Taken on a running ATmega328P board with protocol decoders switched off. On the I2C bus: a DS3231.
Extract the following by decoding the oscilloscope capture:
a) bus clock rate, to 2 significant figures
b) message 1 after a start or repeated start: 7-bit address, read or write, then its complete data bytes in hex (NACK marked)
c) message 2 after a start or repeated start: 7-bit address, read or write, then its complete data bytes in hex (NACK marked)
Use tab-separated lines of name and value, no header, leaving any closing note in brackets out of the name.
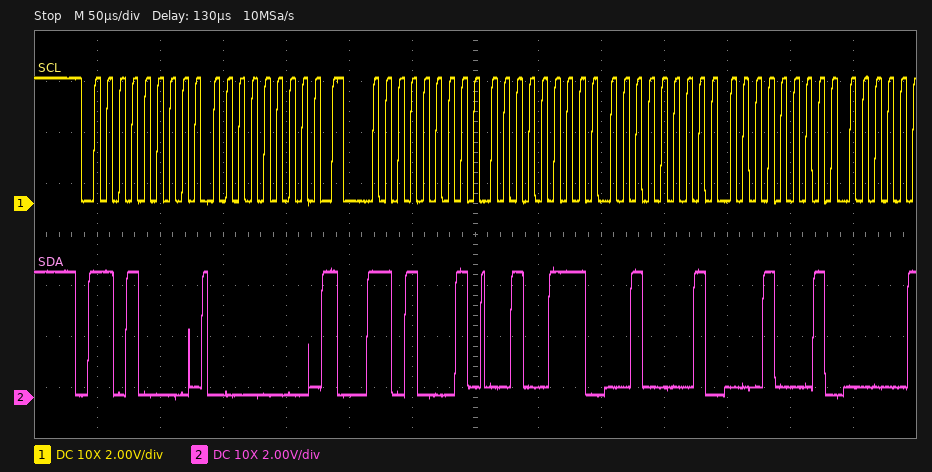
bus clock rate, to 2 significant figures	100 kHz
message 1 after a start or repeated start: 7-bit address, read or write, then its complete data bytes in hex	0x68 write: 00
message 2 after a start or repeated start: 7-bit address, read or write, then its complete data bytes in hex	0x68 read: 27 21 11
